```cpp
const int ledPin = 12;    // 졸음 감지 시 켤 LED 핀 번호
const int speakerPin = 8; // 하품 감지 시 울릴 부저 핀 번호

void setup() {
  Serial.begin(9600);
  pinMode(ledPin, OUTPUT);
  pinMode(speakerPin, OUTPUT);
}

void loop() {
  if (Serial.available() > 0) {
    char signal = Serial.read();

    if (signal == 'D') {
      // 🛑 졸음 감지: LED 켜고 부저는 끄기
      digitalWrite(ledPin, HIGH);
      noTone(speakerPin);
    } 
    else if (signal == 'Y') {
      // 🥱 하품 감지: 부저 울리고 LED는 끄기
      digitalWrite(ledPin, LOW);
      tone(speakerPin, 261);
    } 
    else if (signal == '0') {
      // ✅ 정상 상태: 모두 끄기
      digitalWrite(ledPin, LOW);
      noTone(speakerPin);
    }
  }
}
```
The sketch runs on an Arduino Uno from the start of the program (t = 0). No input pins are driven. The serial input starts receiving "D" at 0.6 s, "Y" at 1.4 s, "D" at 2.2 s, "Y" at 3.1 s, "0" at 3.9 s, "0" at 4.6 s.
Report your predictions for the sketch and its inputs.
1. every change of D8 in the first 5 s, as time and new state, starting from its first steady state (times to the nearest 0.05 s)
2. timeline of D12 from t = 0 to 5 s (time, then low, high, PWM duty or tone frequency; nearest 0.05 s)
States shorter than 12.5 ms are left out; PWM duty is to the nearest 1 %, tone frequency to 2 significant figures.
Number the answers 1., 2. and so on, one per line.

1. 0 s low; 1.4 s tone 260 Hz; 2.2 s low; 3.1 s tone 260 Hz; 3.9 s low
2. 0 s low; 0.6 s high; 1.4 s low; 2.2 s high; 3.1 s low
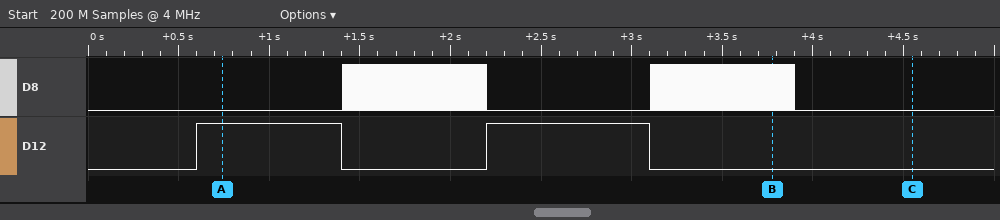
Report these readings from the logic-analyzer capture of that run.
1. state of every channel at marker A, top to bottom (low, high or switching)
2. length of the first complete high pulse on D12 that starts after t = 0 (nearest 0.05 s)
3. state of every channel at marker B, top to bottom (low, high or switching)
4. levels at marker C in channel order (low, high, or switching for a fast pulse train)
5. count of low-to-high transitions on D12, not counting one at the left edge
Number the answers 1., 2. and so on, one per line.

1. D8 low, D12 high
2. 0.80 s
3. D8 switching, D12 low
4. D8 low, D12 low
5. 2
